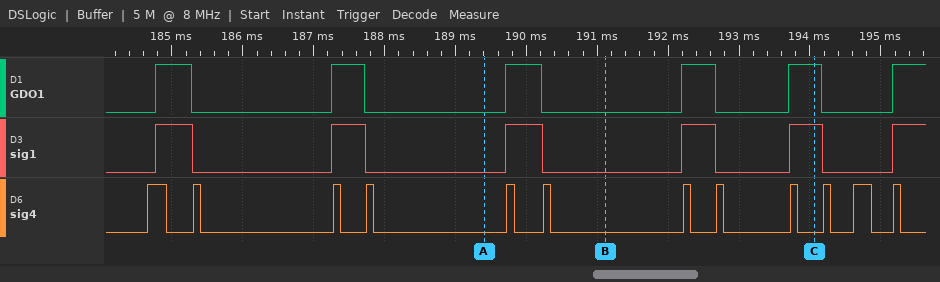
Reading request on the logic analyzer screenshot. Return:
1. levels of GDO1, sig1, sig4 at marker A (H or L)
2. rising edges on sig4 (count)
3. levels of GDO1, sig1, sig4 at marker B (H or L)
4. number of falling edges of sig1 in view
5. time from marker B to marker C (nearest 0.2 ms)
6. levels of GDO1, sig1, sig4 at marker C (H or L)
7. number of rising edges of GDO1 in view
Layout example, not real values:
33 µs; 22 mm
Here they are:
GDO1=L, sig1=L, sig4=L; 12; GDO1=L, sig1=L, sig4=L; 5; 3 ms; GDO1=H, sig1=H, sig4=L; 6
